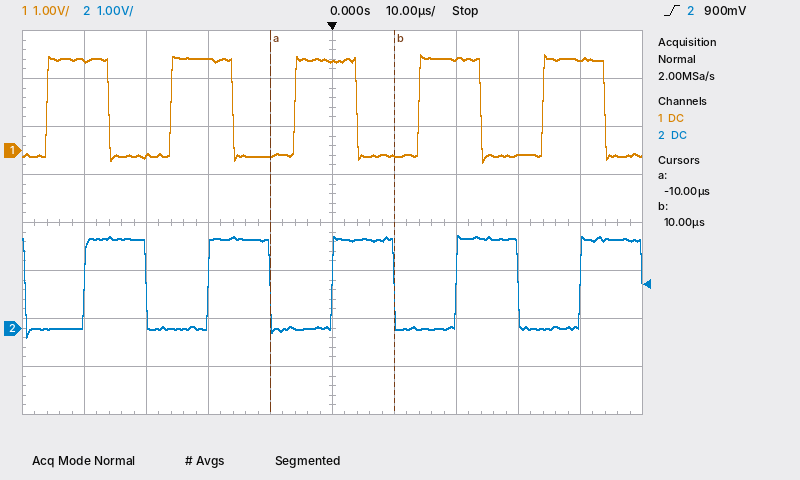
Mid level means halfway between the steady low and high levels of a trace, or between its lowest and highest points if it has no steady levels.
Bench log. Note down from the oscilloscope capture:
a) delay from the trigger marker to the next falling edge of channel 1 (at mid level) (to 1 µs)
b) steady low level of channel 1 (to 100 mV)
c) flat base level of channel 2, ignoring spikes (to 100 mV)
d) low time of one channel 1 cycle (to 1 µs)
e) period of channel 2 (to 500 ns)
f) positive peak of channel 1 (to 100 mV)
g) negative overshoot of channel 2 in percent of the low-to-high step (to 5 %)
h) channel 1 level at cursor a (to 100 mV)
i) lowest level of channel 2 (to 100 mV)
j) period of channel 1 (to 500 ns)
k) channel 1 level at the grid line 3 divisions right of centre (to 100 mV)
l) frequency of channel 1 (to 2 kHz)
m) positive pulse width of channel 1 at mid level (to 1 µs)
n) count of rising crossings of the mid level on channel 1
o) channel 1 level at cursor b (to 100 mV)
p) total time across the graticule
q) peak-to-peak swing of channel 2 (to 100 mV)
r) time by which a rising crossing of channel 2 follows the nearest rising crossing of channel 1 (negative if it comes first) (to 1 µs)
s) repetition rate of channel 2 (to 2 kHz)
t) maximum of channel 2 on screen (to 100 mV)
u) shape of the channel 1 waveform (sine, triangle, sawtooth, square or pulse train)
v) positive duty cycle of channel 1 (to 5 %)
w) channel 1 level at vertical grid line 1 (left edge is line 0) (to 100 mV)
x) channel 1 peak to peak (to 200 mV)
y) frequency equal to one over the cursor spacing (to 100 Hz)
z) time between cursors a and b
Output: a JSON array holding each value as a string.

["4 µs", "-100 mV", "0.0 V", "10 µs", "20.0 µs", "2.0 V", "10 %", "-100 mV", "-200 mV", "20.0 µs", "-100 mV", "50 kHz", "10 µs", "5", "-100 mV", "100 µs", "2.1 V", "+6 µs", "50 kHz", "1.9 V", "square", "50 %", "1.9 V", "2.2 V", "50.0 kHz", "20 µs"]
